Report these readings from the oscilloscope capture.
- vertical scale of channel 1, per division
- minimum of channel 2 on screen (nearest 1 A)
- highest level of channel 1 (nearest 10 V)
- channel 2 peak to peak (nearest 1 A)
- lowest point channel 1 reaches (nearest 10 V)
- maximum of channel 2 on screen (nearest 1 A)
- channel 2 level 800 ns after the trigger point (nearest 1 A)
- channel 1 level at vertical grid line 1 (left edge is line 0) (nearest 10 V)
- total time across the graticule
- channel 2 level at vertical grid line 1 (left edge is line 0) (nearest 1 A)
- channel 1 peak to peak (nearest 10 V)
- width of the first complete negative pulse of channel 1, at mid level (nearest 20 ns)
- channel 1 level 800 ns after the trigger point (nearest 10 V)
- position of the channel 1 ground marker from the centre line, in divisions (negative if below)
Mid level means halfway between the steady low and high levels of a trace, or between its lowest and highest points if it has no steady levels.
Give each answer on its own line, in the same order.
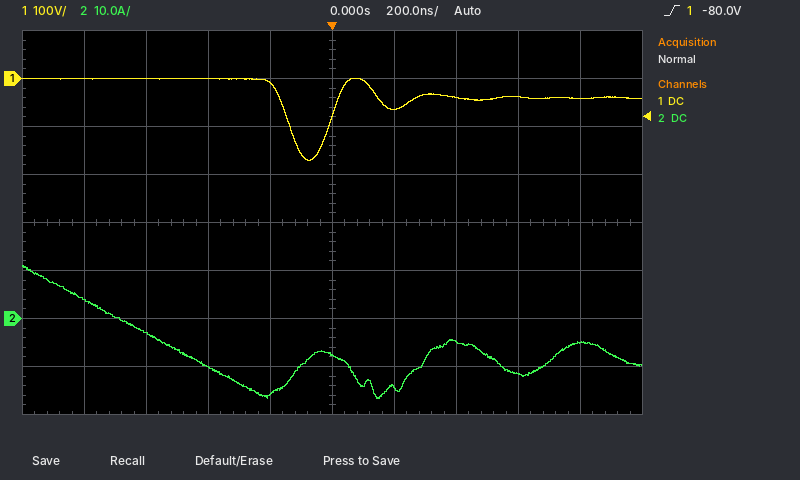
100 V
-17 A
0 V
28 A
-170 V
11 A
-5 A
0 V
2 µs
4 A
170 V
140 ns
-40 V
+3.0 div
